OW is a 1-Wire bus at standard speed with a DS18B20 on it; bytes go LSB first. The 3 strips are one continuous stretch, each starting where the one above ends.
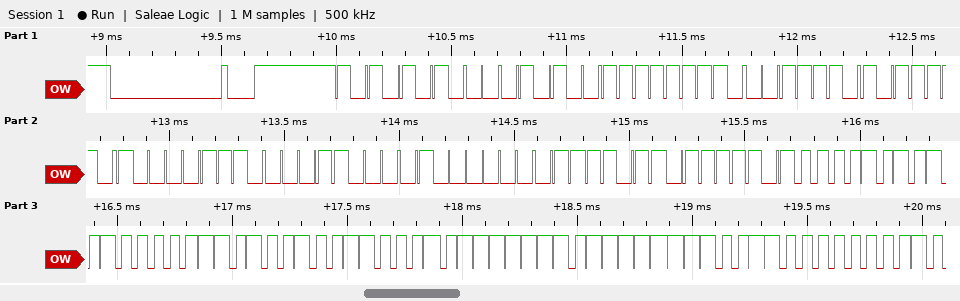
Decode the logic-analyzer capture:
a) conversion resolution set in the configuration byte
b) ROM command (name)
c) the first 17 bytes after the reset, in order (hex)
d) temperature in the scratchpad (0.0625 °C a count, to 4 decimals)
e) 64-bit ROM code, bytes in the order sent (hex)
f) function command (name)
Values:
12 bits
Match ROM
55 28 FF 78 BD 70 18 02 DE BE 50 05 4B 46 7F FF 0C
85.0000 °C
28 FF 78 BD 70 18 02 DE
Read Scratchpad
